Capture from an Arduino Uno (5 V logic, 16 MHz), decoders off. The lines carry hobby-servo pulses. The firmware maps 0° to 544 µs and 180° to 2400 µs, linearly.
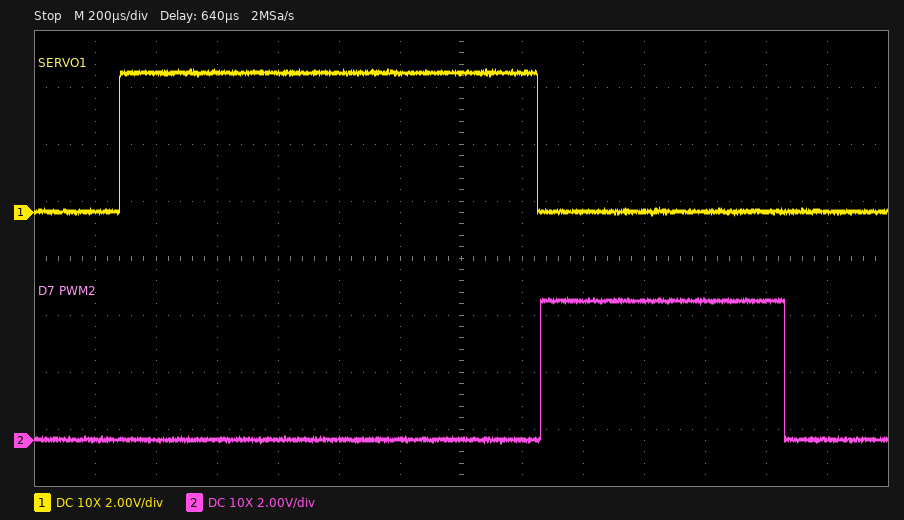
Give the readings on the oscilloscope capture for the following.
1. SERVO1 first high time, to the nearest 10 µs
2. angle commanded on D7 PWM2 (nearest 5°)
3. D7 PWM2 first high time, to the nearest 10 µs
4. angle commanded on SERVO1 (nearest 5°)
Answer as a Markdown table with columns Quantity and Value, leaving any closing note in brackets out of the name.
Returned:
| Quantity | Value |
|---|---|
| SERVO1 first high time, to the nearest 10 µs | 1370 µs |
| angle commanded on D7 PWM2 | 25° |
| D7 PWM2 first high time, to the nearest 10 µs | 800 µs |
| angle commanded on SERVO1 | 80° |
